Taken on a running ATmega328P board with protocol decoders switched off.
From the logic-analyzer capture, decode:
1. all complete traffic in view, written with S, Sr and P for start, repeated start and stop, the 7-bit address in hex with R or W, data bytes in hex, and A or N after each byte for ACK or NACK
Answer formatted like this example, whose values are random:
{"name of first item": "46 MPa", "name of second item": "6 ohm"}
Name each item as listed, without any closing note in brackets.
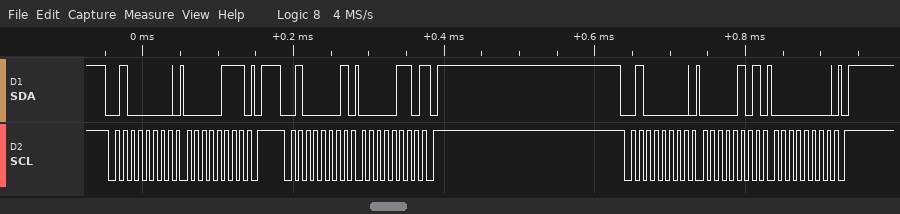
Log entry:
{"all complete traffic in view, written with S, Sr and P for start, repeated start and stop, the 7-bit address in hex with R or W, data bytes in hex, and A or N after each byte for ACK or NACK": "S 20W A 07 A P S 20R A 06 N P S 20W A 05 A 00 A P"}
